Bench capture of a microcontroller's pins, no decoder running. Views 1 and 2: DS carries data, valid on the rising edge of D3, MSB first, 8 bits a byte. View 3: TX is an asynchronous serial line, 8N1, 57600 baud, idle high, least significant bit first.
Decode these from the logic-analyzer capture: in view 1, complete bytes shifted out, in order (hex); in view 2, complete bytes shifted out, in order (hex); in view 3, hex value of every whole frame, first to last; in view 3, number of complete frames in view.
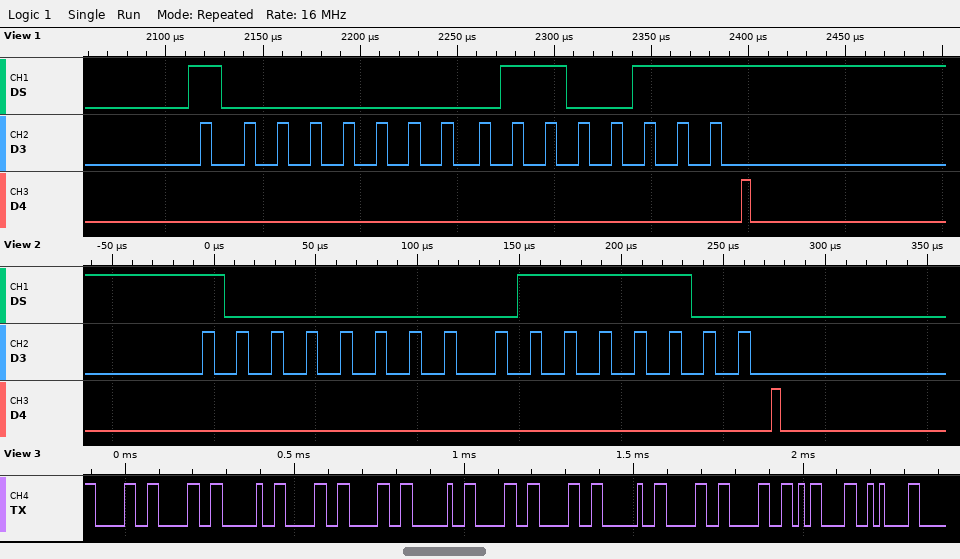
80 67
80 7C
30 30 20 30 30 20 30 30 20 30 30 0D 0A
13
